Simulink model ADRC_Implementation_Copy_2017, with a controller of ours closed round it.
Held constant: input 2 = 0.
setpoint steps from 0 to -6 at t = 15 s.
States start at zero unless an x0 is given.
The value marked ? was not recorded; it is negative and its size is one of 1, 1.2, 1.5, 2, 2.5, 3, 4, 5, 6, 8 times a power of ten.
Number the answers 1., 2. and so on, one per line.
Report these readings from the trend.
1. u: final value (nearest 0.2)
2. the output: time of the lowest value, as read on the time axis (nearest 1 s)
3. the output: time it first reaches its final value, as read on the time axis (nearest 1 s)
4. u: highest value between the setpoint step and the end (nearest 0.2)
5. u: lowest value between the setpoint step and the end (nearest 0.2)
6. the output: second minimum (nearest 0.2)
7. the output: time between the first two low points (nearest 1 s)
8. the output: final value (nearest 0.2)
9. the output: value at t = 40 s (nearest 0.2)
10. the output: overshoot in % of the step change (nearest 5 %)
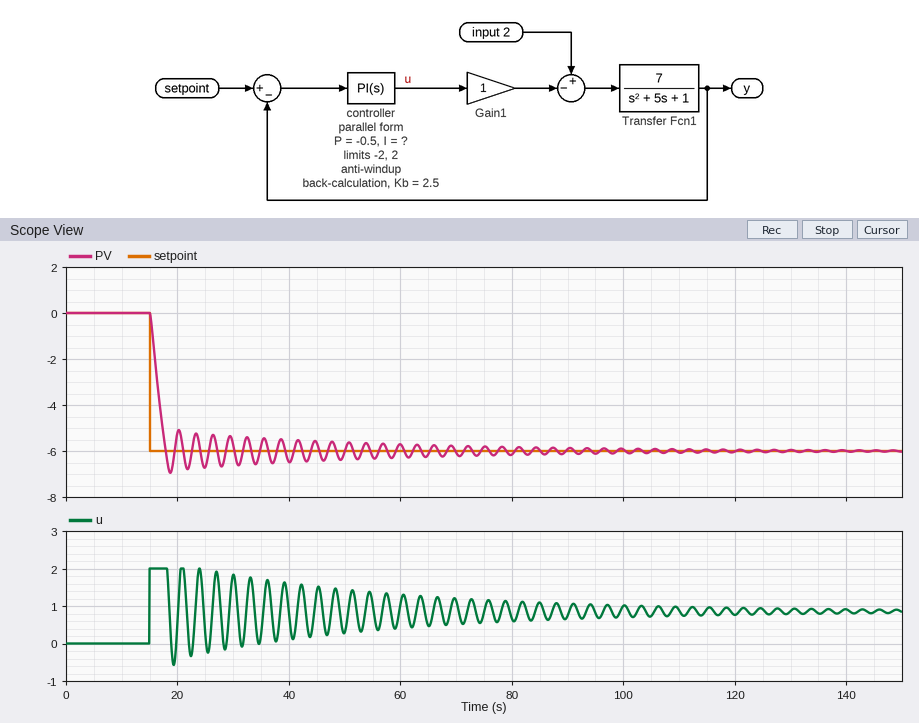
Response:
1. 0.8
2. 19 s
3. 18 s
4. 2.0
5. -0.6
6. -6.8
7. 3 s
8. -6.0
9. -6.4
10. 15 %
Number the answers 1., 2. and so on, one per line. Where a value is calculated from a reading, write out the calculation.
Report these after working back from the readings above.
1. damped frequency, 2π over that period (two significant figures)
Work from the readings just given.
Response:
1. 2π / 3 = 2.1 rad/s
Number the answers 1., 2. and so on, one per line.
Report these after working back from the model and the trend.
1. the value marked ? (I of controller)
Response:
1. -3
